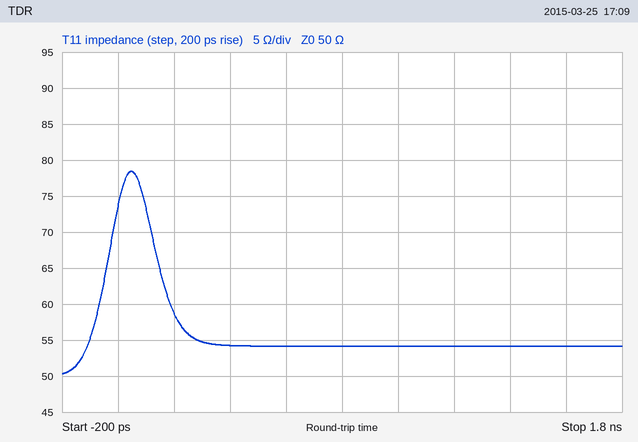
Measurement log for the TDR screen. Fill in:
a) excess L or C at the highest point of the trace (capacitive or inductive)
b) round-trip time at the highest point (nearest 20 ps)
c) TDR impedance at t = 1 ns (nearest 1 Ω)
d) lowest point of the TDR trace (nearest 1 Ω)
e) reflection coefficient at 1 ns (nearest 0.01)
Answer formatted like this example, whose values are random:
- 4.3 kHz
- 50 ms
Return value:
- inductive
- 40 ps
- 54 Ω
- 50 Ω
- +0.04
